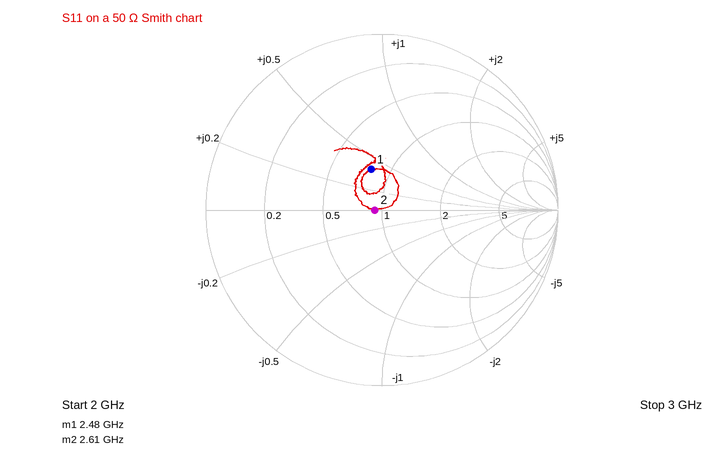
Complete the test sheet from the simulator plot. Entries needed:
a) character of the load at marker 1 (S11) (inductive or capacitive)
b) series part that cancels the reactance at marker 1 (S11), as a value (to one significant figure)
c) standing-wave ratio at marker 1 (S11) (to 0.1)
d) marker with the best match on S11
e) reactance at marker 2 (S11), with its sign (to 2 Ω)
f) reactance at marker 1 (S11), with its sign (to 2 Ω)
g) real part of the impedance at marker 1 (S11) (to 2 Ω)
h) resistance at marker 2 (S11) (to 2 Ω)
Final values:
inductive
3 pF
1.6
marker 2
0 Ω
+20 Ω
40 Ω
46 Ω
